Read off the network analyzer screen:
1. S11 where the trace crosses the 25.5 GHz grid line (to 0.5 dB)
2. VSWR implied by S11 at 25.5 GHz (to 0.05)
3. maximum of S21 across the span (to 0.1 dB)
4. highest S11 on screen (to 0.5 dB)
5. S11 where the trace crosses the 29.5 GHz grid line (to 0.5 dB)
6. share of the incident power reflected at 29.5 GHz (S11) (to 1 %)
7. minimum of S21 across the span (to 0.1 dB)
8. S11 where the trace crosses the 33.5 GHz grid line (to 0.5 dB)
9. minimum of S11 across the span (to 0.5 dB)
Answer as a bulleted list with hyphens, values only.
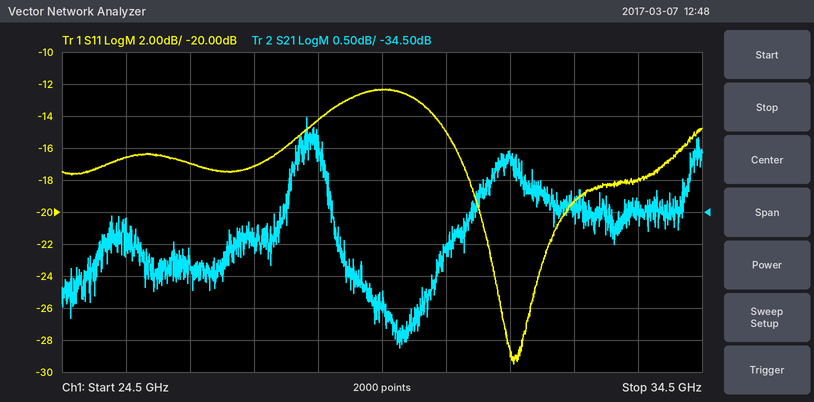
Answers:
- -16.5 dB
- 1.35
- -33.0 dB
- -12.5 dB
- -12.5 dB
- 6 %
- -36.6 dB
- -18.0 dB
- -29.5 dB
